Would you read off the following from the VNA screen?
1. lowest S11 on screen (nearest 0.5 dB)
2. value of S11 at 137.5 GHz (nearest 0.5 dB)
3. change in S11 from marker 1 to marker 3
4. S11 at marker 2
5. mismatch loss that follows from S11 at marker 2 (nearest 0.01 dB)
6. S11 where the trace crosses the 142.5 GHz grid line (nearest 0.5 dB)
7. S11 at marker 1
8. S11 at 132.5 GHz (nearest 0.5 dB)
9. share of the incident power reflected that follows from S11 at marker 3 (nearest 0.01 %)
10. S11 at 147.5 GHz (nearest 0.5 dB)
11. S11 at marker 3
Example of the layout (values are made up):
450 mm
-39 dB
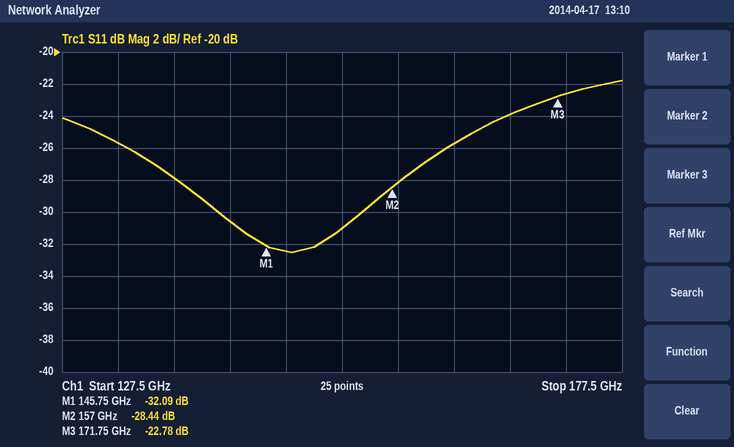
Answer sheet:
-32.5 dB
-28.0 dB
9.31 dB
-28.44 dB
0.01 dB
-30.5 dB
-32.09 dB
-25.5 dB
0.53 %
-32.5 dB
-22.78 dB
